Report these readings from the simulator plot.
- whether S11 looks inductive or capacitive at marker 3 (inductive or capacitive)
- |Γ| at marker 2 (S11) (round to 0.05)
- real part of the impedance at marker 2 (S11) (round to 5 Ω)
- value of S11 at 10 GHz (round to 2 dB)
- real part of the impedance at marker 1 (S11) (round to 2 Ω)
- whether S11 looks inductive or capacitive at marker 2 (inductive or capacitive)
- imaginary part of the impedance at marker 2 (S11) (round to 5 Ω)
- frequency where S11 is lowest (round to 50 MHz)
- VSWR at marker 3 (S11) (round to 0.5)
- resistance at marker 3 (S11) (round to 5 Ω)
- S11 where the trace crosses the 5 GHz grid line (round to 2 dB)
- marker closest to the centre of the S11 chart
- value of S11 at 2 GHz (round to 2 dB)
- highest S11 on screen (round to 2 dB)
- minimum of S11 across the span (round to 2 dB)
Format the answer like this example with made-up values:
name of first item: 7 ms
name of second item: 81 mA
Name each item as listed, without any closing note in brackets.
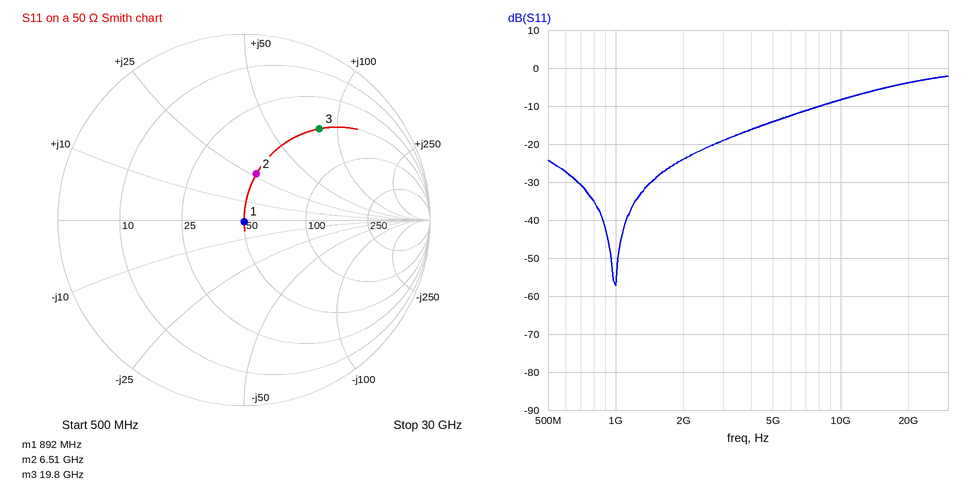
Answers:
whether S11 looks inductive or capacitive at marker 3: inductive
|Γ| at marker 2 (S11): 0.25
real part of the impedance at marker 2 (S11): 50 Ω
value of S11 at 10 GHz: -8 dB
real part of the impedance at marker 1 (S11): 50 Ω
whether S11 looks inductive or capacitive at marker 2: inductive
imaginary part of the impedance at marker 2 (S11): +25 Ω
frequency where S11 is lowest: 1.00 GHz
VSWR at marker 3 (S11): 4.5
resistance at marker 3 (S11): 50 Ω
S11 where the trace crosses the 5 GHz grid line: -14 dB
marker closest to the centre of the S11 chart: marker 1
value of S11 at 2 GHz: -24 dB
highest S11 on screen: -2 dB
minimum of S11 across the span: -58 dB
